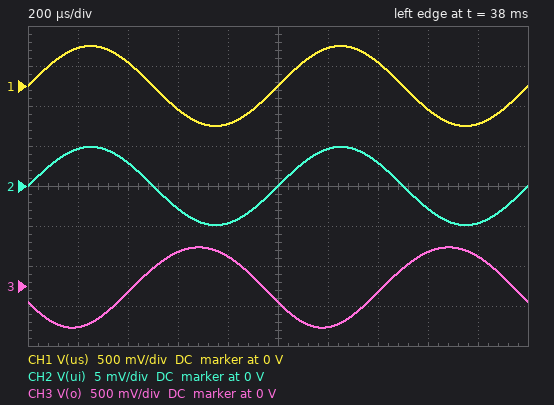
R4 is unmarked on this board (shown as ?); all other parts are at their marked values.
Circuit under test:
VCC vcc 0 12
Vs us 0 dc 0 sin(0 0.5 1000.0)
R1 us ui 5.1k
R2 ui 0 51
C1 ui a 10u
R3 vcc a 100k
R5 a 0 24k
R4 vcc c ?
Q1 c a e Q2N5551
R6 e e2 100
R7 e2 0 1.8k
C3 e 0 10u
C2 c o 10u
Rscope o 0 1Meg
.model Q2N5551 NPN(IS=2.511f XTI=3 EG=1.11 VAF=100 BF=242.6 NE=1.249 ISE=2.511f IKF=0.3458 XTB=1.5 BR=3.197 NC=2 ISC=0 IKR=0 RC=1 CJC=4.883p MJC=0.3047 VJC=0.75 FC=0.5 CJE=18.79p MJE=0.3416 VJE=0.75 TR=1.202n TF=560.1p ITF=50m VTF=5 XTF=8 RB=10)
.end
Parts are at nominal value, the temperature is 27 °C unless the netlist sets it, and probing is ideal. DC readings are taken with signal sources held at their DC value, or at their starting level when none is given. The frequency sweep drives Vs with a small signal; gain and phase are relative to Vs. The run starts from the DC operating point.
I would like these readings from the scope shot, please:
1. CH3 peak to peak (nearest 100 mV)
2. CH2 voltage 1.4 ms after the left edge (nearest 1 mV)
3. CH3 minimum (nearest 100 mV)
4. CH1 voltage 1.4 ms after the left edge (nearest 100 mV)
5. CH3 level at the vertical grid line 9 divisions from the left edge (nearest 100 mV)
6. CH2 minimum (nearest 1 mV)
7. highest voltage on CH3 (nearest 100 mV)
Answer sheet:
1.0 V
3 mV
-500 mV
300 mV
400 mV
-5 mV
500 mV
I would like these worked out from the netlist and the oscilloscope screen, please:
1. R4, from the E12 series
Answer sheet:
3.9 kΩ
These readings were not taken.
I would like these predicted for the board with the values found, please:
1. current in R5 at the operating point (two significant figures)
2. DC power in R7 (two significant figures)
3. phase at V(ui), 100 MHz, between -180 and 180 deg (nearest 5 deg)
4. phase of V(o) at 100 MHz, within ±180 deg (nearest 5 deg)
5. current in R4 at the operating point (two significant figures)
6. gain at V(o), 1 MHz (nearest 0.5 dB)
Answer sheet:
91 µA
1.1 mW
-20 deg
60 deg
790 µA
1.0 dB
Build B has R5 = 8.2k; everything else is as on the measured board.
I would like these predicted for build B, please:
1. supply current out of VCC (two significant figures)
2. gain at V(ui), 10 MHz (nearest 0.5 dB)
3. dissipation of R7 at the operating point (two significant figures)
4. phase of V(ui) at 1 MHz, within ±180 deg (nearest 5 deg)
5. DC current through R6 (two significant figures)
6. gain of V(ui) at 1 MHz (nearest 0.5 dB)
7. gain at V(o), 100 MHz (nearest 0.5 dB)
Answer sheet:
250 µA
-41.0 dB
34 µW
0 deg
140 µA
-40.0 dB
-33.5 dB
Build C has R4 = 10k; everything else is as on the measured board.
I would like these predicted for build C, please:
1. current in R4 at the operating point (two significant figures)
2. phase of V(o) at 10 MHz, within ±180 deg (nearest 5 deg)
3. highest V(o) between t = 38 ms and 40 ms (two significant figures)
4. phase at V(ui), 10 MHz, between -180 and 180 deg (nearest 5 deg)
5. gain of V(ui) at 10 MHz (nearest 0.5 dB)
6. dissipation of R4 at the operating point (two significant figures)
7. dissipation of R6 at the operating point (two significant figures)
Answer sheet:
780 µA
95 deg
1.2 V
-15 deg
-46.5 dB
6.1 mW
62 µW
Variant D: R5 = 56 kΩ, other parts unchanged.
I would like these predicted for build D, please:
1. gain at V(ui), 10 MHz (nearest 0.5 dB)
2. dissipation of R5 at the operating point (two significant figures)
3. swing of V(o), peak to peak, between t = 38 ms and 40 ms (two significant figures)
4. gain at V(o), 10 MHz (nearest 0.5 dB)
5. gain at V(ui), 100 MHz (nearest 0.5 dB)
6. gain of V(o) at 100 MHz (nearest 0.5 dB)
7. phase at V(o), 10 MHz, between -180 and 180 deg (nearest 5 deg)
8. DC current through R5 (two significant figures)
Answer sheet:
-48.0 dB
260 µW
1.6 V
-5.0 dB
-50.5 dB
-25.5 dB
100 deg
68 µA
